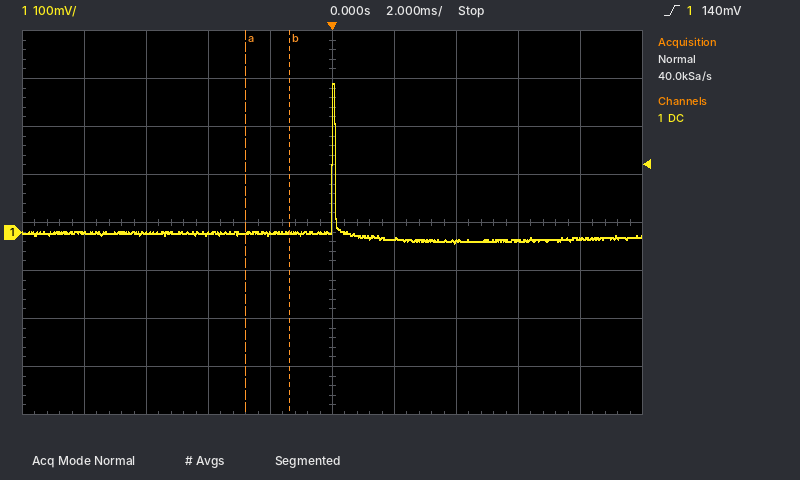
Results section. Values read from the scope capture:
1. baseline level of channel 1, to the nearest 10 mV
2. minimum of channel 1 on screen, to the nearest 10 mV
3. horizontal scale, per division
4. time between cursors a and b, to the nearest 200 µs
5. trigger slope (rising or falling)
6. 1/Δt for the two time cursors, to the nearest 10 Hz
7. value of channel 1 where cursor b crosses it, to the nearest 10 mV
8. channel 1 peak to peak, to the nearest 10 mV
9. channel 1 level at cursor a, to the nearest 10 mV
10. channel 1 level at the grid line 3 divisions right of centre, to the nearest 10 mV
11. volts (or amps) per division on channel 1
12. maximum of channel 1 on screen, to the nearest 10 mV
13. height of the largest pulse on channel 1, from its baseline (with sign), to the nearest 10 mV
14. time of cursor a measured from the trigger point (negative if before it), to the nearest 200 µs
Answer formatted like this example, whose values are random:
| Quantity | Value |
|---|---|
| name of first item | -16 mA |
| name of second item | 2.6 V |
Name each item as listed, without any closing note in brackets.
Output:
| Quantity | Value |
|---|---|
| baseline level of channel 1, to the nearest 10 mV | 0 mV |
| minimum of channel 1 on screen, to the nearest 10 mV | -20 mV |
| horizontal scale, per division | 2 ms |
| time between cursors a and b, to the nearest 200 µs | 1.4 ms |
| trigger slope | rising |
| 1/Δt for the two time cursors, to the nearest 10 Hz | 710 Hz |
| value of channel 1 where cursor b crosses it, to the nearest 10 mV | 0 mV |
| channel 1 peak to peak, to the nearest 10 mV | 330 mV |
| channel 1 level at cursor a, to the nearest 10 mV | 0 mV |
| channel 1 level at the grid line 3 divisions right of centre, to the nearest 10 mV | -20 mV |
| volts (or amps) per division on channel 1 | 100 mV |
| maximum of channel 1 on screen, to the nearest 10 mV | 310 mV |
| height of the largest pulse on channel 1, from its baseline (with sign), to the nearest 10 mV | +310 mV |
| time of cursor a measured from the trigger point (negative if before it), to the nearest 200 µs | -2.8 ms |
